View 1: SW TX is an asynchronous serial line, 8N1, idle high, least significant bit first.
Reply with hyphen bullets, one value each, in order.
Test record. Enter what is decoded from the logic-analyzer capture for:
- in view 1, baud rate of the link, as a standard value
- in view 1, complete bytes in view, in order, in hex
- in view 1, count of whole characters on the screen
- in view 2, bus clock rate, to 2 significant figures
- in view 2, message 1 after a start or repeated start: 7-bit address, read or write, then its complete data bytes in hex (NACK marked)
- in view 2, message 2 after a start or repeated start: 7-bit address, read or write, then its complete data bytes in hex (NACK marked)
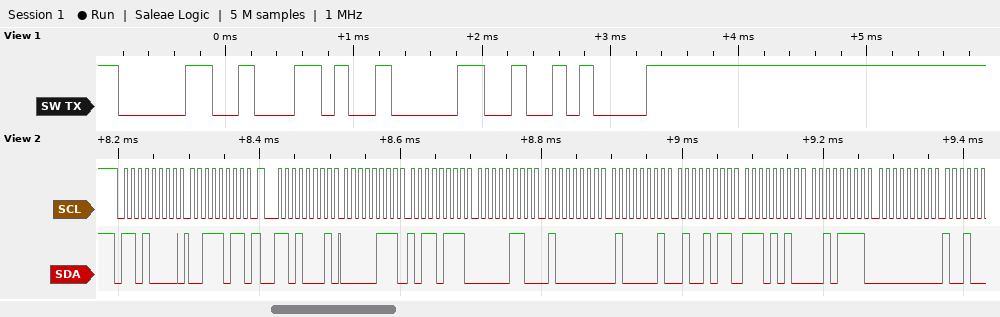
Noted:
- 9600 baud
- 30 2C 30 0A
- 4
- 100 kHz
- 0x68 write: 3B
- 0x68 read: 07 B7 06 40 41 4B EA 2F 00
